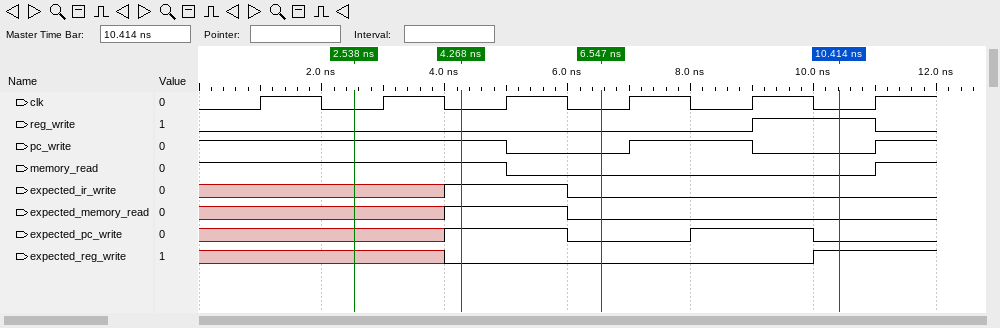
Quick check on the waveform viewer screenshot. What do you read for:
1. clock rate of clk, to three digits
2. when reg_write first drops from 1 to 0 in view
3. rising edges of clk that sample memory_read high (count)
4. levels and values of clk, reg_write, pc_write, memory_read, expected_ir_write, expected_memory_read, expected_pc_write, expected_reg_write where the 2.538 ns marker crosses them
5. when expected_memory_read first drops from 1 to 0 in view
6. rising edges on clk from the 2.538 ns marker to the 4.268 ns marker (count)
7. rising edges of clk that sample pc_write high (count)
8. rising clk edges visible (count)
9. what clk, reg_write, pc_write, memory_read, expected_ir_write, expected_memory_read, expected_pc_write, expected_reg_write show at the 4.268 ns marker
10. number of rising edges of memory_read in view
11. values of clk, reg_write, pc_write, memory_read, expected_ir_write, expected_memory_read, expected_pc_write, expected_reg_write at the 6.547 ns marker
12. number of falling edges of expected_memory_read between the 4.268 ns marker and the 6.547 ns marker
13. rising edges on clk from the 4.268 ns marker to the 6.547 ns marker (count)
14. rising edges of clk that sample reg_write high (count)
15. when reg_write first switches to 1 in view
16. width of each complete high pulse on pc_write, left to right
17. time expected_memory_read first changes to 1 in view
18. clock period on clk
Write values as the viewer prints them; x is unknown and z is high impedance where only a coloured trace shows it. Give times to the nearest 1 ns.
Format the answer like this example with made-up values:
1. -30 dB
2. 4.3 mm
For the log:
1. 500 MHz
2. 11 ns
3. 3
4. clk=0, reg_write=0, pc_write=1, memory_read=1, expected_ir_write=x, expected_memory_read=x, expected_pc_write=x, expected_reg_write=x
5. 6 ns
6. 1
7. 4
8. 6
9. clk=0, reg_write=0, pc_write=1, memory_read=1, expected_ir_write=1, expected_memory_read=1, expected_pc_write=1, expected_reg_write=0
10. 1
11. clk=0, reg_write=0, pc_write=0, memory_read=0, expected_ir_write=0, expected_memory_read=0, expected_pc_write=0, expected_reg_write=0
12. 1
13. 1
14. 1
15. 9 ns
16. 2 ns
17. 4 ns
18. 2 ns
